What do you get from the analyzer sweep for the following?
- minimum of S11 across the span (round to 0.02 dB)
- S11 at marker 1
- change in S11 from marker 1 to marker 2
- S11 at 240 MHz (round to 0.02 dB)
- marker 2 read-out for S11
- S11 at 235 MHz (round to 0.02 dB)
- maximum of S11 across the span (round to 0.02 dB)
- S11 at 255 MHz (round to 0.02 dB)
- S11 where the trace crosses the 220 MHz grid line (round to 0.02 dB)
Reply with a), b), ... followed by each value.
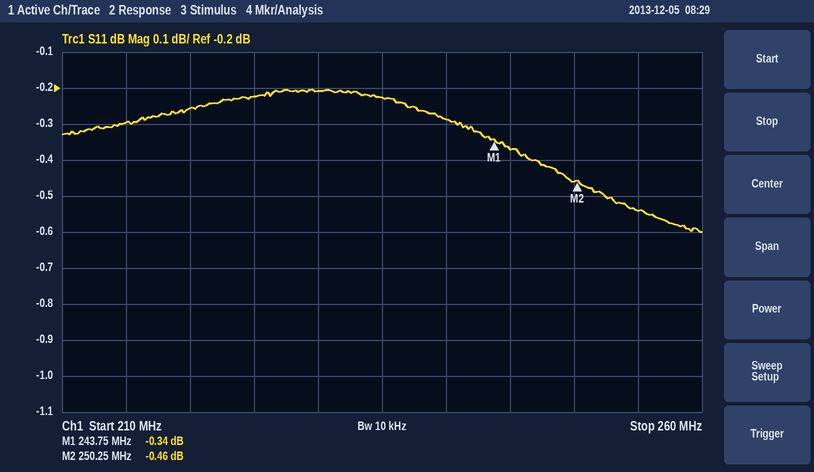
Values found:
a) -0.60 dB
b) -0.34 dB
c) -0.12 dB
d) -0.28 dB
e) -0.46 dB
f) -0.22 dB
g) -0.20 dB
h) -0.54 dB
i) -0.26 dB
